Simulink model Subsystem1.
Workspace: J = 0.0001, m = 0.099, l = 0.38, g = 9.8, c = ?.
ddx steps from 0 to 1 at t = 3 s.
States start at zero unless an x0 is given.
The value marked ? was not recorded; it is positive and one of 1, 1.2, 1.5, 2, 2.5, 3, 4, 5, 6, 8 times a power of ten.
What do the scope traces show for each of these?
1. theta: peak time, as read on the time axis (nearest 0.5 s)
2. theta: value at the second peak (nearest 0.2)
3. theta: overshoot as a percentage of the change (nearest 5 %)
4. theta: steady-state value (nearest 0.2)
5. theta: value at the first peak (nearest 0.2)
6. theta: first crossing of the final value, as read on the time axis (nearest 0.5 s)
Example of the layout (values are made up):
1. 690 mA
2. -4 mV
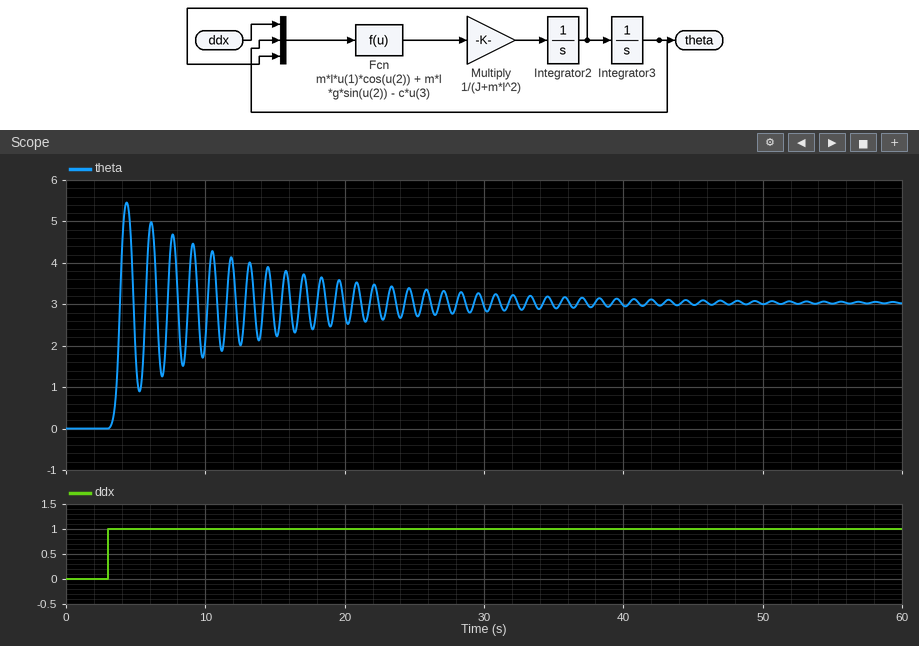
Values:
1. 4.5 s
2. 5.0
3. 80 %
4. 3.0
5. 5.4
6. 4.0 s
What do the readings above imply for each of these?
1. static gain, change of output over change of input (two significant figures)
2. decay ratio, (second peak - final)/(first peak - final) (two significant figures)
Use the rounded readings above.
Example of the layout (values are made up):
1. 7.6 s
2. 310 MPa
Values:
1. 3.0
2. 0.83
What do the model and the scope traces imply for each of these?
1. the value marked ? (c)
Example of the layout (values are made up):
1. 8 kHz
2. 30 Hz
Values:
1. 0.0025
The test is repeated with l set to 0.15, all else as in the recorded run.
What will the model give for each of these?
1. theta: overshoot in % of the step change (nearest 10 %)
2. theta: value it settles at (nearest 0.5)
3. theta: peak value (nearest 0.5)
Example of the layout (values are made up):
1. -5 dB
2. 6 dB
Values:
1. 60 %
2. 3.0
3. 5.0
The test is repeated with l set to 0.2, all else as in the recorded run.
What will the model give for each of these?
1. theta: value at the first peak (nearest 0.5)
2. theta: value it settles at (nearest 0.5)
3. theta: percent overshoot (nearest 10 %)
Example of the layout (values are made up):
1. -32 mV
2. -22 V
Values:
1. 5.0
2. 3.0
3. 70 %
